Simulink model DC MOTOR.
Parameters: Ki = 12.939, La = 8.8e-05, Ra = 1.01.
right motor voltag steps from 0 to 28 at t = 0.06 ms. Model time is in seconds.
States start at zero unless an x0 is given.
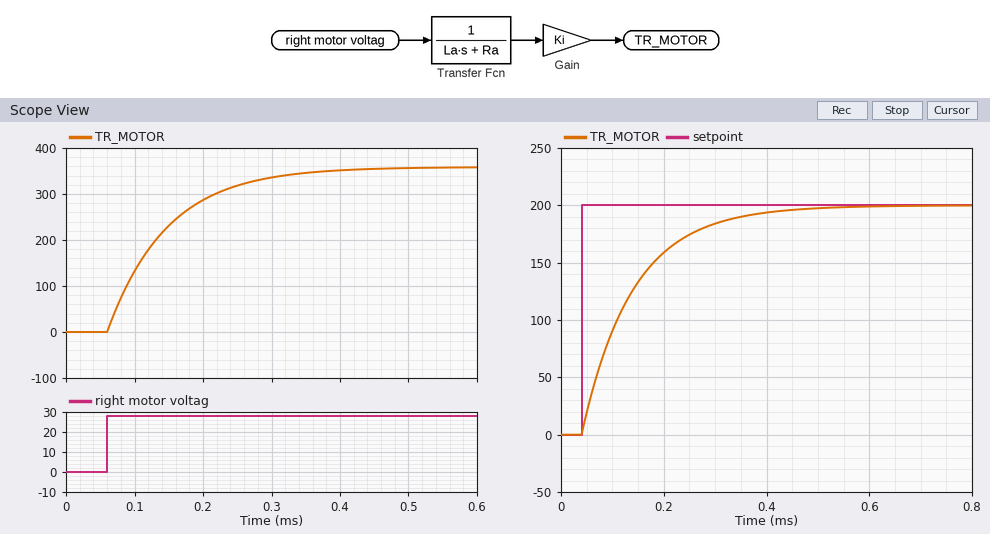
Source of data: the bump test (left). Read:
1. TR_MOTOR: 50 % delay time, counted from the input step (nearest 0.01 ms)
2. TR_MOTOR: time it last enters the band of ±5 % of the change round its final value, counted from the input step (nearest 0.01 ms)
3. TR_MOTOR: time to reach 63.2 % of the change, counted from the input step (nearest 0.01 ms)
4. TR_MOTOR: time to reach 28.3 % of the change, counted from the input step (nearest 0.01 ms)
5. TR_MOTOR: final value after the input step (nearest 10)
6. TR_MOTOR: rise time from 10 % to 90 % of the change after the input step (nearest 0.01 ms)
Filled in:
0.06 ms
0.26 ms
0.09 ms
0.03 ms
360
0.19 ms
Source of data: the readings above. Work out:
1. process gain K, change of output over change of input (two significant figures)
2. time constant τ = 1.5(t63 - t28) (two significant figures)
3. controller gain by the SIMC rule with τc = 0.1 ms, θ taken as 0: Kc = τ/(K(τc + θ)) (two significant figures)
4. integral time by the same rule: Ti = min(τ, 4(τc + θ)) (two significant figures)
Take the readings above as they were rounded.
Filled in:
13
0.090 ms
0.069
0.090 ms
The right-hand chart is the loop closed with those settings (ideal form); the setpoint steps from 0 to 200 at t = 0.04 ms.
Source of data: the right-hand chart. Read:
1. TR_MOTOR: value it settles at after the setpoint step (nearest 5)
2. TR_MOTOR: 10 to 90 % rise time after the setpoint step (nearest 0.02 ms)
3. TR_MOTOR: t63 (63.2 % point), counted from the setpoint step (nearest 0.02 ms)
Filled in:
200
0.22 ms
0.10 ms
